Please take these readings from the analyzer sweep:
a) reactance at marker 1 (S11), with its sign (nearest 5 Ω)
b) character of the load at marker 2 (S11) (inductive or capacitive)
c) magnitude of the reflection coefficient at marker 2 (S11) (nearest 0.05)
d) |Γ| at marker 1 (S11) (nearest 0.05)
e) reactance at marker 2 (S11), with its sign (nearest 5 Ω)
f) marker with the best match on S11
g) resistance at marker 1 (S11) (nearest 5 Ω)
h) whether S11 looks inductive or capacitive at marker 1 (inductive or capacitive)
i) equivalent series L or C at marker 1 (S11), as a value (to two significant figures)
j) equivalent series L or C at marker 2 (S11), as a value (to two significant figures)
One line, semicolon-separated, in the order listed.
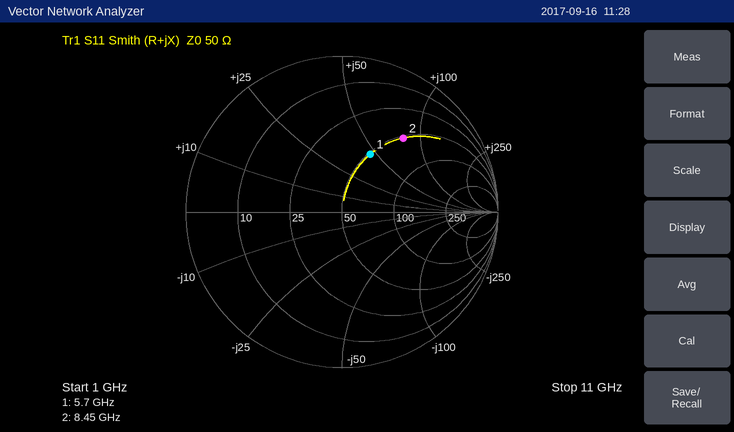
+45 Ω; inductive; 0.60; 0.40; +80 Ω; marker 1; 50 Ω; inductive; 1.3 nH; 1.5 nH
